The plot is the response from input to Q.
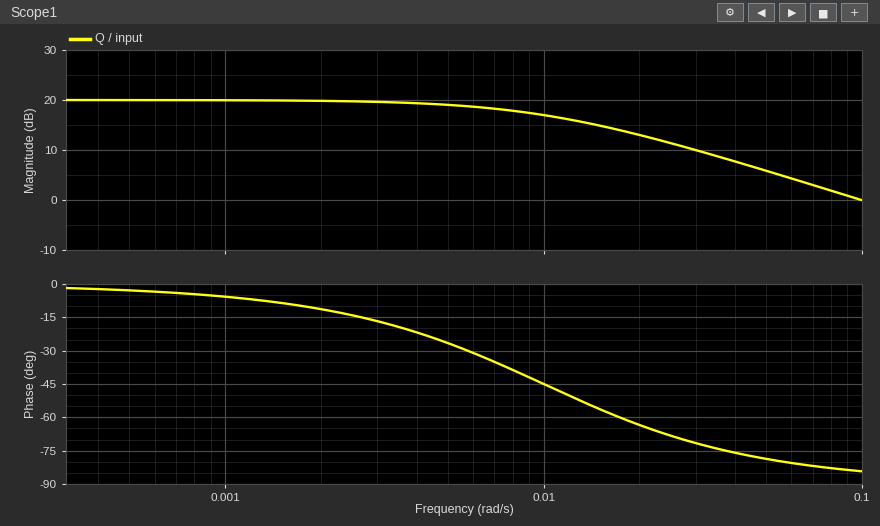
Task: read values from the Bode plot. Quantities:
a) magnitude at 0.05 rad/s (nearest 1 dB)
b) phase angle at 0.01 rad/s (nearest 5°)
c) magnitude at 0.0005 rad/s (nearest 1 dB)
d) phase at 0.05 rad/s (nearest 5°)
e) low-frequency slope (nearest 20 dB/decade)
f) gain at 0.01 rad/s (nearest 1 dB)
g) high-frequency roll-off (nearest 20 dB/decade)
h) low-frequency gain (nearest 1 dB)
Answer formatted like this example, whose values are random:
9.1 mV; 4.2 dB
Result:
6 dB; -45°; 20 dB; -80°; 0 dB/decade; 17 dB; -20 dB/decade; 20 dB
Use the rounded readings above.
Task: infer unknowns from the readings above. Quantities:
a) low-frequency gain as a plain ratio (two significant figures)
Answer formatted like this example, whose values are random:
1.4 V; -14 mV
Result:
10
